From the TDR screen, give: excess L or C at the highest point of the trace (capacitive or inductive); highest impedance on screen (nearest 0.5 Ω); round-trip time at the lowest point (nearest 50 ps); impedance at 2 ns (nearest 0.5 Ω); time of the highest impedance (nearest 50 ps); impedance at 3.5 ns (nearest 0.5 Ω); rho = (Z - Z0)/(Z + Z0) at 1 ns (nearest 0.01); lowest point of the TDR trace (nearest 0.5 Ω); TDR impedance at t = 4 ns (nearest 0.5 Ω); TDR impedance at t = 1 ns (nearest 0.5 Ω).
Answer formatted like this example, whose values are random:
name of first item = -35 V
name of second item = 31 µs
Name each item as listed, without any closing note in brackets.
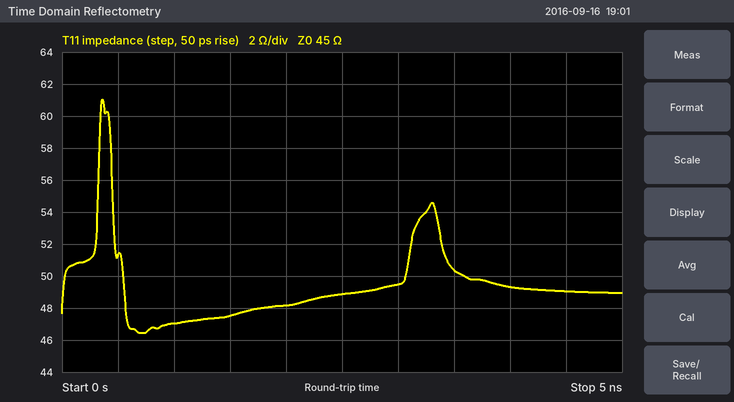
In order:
excess L or C at the highest point of the trace = inductive
highest impedance on screen = 61.0 Ω
round-trip time at the lowest point = 700 ps
impedance at 2 ns = 48.0 Ω
time of the highest impedance = 350 ps
impedance at 3.5 ns = 50.5 Ω
rho = (Z - Z0)/(Z + Z0) at 1 ns = +0.02
lowest point of the TDR trace = 46.5 Ω
TDR impedance at t = 4 ns = 49.5 Ω
TDR impedance at t = 1 ns = 47.0 Ω
